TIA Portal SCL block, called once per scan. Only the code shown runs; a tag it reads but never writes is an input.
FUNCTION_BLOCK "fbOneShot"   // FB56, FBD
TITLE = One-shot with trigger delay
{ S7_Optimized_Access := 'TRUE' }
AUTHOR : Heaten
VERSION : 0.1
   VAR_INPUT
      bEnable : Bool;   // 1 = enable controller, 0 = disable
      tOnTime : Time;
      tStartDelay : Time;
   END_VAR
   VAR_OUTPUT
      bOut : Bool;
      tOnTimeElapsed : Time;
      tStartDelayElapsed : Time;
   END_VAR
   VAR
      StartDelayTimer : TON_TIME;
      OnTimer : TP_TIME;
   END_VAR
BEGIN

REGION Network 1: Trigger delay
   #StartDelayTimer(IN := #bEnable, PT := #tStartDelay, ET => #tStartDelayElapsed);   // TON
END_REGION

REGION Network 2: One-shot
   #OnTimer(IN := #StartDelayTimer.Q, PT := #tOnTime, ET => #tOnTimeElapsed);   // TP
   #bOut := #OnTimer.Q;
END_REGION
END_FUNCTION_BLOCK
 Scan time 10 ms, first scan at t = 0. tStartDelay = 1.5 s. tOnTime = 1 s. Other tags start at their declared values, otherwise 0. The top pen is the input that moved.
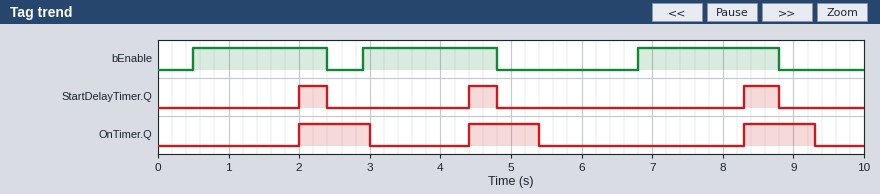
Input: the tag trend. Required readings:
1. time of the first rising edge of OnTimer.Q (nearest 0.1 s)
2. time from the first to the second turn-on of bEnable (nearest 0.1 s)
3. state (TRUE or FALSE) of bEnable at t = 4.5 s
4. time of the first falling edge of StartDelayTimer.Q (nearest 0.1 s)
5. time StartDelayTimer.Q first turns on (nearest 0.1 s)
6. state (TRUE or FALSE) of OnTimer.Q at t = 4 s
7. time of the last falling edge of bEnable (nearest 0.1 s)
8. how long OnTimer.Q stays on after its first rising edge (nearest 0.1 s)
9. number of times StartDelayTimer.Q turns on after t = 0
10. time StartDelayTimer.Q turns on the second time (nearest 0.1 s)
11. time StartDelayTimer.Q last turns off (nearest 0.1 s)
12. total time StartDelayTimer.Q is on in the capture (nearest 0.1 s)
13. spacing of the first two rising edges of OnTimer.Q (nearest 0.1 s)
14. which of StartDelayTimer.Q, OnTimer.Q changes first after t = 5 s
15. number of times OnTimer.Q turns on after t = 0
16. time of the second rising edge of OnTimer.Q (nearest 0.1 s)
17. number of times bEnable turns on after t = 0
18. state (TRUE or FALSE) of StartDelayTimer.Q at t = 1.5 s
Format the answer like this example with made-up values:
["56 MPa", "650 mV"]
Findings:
["2.0 s", "2.4 s", "TRUE", "2.4 s", "2.0 s", "FALSE", "8.8 s", "1.0 s", "3", "4.4 s", "8.8 s", "1.3 s", "2.4 s", "OnTimer.Q", "3", "4.4 s", "3", "FALSE"]
